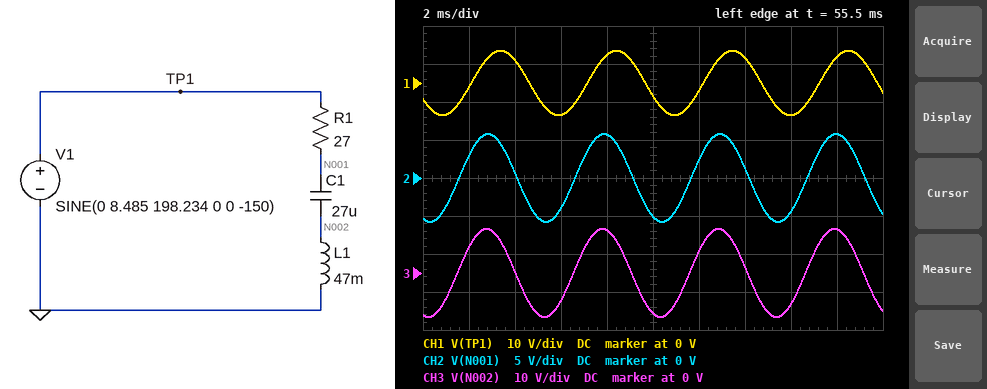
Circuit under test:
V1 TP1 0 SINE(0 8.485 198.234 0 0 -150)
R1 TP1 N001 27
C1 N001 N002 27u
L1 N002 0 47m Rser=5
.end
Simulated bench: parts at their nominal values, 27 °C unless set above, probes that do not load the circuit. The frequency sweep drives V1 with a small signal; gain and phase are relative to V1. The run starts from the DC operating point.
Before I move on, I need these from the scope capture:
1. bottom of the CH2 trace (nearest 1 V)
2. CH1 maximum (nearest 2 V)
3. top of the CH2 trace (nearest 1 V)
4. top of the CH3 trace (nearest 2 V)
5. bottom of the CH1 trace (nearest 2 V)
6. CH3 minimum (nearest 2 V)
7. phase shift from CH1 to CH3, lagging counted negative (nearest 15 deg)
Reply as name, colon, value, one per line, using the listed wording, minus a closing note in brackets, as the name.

bottom of the CH2 trace: -6 V
CH1 maximum: 8 V
top of the CH2 trace: 6 V
top of the CH3 trace: 12 V
bottom of the CH1 trace: -8 V
CH3 minimum: -12 V
phase shift from CH1 to CH3, lagging counted negative: 45 deg
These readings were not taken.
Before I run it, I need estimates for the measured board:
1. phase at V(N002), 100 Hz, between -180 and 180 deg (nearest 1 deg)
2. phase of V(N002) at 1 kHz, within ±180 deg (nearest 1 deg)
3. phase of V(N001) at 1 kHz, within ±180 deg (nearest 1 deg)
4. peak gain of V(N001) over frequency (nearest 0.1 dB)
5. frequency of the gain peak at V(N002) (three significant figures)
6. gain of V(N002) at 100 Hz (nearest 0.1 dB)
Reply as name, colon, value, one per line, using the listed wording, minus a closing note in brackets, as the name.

phase at V(N002), 100 Hz, between -180 and 180 deg: 123 deg
phase of V(N002) at 1 kHz, within ±180 deg: 5 deg
phase of V(N001) at 1 kHz, within ±180 deg: 5 deg
peak gain of V(N001) over frequency: 0 dB
frequency of the gain peak at V(N002): 168 Hz
gain of V(N002) at 100 Hz: -3.2 dB
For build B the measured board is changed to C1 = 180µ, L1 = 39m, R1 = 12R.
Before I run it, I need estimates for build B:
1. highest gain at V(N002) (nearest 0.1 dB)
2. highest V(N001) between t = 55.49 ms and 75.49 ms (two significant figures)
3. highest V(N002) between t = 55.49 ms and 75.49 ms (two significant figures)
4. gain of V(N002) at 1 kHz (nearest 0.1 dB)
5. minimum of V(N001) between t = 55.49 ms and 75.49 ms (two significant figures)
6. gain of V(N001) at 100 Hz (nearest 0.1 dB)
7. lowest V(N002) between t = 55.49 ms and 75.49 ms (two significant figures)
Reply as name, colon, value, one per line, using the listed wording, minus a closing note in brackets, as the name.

highest gain at V(N002): 0.7 dB
highest V(N001) between t = 55.49 ms and 75.49 ms: 8.0 V
highest V(N002) between t = 55.49 ms and 75.49 ms: 8.8 V
gain of V(N002) at 1 kHz: 0 dB
minimum of V(N001) between t = 55.49 ms and 75.49 ms: -8.0 V
gain of V(N001) at 100 Hz: -3.0 dB
lowest V(N002) between t = 55.49 ms and 75.49 ms: -8.8 V
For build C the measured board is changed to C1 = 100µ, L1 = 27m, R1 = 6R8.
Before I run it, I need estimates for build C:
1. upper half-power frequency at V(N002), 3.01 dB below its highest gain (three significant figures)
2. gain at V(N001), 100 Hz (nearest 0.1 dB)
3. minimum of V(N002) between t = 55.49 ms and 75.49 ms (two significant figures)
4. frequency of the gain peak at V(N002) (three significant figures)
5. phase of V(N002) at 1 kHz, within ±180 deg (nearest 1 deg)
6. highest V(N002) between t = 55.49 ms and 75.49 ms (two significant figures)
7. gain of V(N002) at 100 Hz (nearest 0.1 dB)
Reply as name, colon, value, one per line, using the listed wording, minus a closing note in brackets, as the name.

upper half-power frequency at V(N002), 3.01 dB below its highest gain: 292 Hz
gain at V(N001), 100 Hz: -7.3 dB
minimum of V(N002) between t = 55.49 ms and 75.49 ms: -10 V
frequency of the gain peak at V(N002): 111 Hz
phase of V(N002) at 1 kHz, within ±180 deg: 2 deg
highest V(N002) between t = 55.49 ms and 75.49 ms: 10 V
gain of V(N002) at 100 Hz: 3.5 dB
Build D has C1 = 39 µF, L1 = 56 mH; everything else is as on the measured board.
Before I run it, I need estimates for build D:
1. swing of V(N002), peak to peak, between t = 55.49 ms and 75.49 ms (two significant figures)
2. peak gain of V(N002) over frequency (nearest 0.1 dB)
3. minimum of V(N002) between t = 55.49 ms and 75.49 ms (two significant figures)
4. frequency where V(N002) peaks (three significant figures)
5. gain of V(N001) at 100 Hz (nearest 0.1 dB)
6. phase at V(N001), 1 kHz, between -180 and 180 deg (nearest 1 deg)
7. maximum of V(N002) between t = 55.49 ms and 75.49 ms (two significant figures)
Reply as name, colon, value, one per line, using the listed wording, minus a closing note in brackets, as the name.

swing of V(N002), peak to peak, between t = 55.49 ms and 75.49 ms: 20 V
peak gain of V(N002) over frequency: 2.4 dB
minimum of V(N002) between t = 55.49 ms and 75.49 ms: -10 V
frequency where V(N002) peaks: 134 Hz
gain of V(N001) at 100 Hz: -12.7 dB
phase at V(N001), 1 kHz, between -180 and 180 deg: 4 deg
maximum of V(N002) between t = 55.49 ms and 75.49 ms: 10 V
